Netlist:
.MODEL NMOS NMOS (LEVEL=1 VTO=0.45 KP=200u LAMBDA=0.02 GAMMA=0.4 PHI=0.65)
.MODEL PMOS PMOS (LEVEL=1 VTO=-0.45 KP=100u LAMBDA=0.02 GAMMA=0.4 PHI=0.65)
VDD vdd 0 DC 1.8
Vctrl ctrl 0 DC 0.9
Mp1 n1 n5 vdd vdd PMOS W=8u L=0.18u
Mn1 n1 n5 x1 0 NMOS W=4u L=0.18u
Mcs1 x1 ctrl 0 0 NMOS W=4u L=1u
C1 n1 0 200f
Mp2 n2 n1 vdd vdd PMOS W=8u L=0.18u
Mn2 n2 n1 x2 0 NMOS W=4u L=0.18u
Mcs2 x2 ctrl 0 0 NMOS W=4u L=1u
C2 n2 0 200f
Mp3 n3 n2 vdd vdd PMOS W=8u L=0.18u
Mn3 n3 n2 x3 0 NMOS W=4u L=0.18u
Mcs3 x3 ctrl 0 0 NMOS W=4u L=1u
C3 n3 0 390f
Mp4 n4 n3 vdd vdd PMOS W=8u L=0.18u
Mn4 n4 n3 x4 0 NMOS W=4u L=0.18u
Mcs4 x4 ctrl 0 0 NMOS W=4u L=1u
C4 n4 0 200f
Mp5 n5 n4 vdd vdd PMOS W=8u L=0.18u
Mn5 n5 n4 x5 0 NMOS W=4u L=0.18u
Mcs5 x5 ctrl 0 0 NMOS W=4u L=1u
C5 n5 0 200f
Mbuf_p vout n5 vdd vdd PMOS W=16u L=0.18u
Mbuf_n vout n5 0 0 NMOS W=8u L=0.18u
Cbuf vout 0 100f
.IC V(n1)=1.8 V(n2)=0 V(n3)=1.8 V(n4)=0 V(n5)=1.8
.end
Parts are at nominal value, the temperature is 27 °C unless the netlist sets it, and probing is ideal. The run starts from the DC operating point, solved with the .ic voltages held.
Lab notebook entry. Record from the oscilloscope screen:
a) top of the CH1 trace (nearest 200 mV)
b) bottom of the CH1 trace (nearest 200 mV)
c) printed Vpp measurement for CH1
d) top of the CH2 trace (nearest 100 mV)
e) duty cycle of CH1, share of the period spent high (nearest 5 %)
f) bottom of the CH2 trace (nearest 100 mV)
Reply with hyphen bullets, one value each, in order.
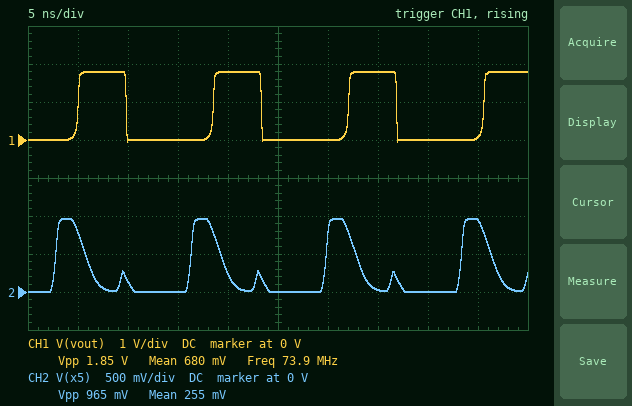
- 1.8 V
- 0 V
- 1.85 V
- 1.0 V
- 35 %
- 0 V
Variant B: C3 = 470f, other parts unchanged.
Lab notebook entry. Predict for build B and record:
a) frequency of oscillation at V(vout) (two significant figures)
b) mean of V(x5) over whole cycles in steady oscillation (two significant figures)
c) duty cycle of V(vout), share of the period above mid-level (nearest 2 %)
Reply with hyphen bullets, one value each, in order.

- 70 MHz
- 230 mV
- 34 %
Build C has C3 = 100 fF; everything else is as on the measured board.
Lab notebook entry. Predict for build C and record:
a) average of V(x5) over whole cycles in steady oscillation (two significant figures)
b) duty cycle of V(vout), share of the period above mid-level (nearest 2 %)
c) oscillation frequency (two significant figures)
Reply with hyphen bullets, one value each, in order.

- 320 mV
- 42 %
- 97 MHz
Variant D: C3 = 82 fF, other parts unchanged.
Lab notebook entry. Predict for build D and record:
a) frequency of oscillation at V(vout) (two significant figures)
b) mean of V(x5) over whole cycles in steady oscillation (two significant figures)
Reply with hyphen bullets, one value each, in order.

- 100 MHz
- 330 mV
